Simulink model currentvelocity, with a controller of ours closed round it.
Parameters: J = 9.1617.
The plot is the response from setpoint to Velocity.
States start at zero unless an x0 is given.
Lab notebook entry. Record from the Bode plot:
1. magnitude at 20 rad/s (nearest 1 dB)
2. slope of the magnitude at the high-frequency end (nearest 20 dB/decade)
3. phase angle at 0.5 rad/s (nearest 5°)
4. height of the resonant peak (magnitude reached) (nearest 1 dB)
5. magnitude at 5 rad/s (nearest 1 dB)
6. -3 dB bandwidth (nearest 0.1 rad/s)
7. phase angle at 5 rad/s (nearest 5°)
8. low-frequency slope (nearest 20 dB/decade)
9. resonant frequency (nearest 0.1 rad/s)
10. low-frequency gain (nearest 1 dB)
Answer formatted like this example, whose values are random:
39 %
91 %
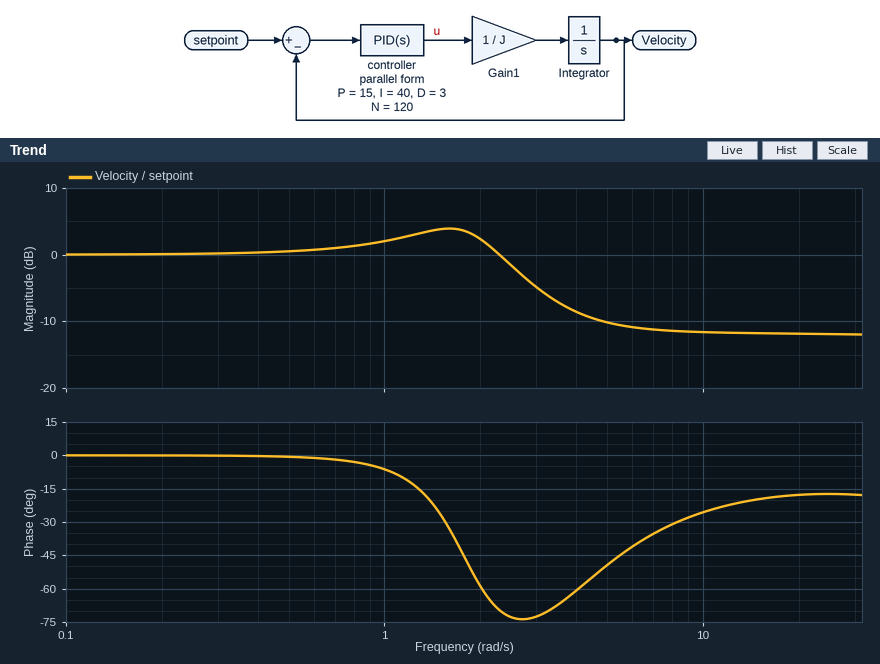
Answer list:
-12 dB
0 dB/decade
0°
4 dB
-10 dB
2.7 rad/s
-50°
0 dB/decade
1.6 rad/s
0 dB
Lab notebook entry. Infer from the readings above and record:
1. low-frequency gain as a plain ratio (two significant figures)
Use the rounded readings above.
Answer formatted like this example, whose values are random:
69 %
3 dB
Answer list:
1.0
